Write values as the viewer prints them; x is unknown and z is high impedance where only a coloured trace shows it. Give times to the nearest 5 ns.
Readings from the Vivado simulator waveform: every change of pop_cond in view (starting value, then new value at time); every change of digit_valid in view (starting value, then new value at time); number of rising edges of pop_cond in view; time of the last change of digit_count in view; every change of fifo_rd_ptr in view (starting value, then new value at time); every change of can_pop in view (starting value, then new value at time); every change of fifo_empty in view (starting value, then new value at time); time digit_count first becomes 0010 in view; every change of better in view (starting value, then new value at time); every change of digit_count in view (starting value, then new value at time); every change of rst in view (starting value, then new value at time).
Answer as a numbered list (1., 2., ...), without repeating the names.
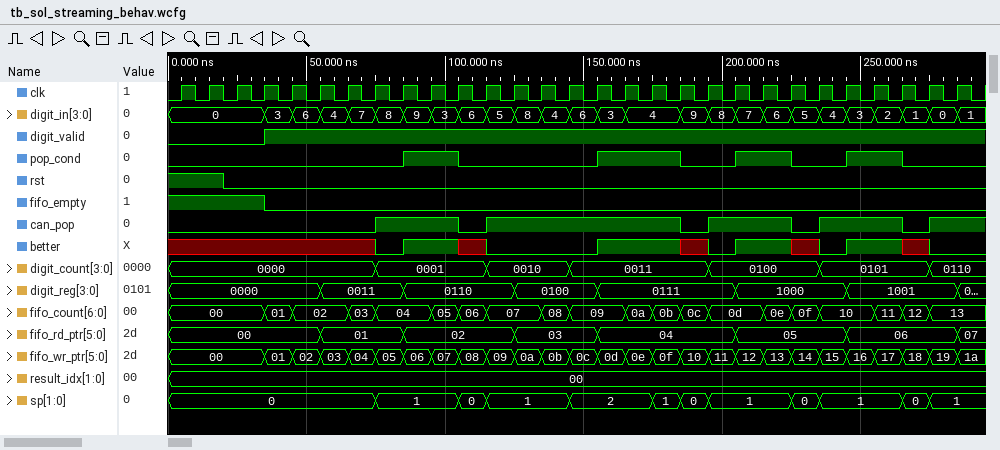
1. 0, 1 at 85 ns, 0 at 105 ns, 1 at 155 ns, 0 at 185 ns, 1 at 205 ns, 0 at 225 ns, 1 at 245 ns, 0 at 265 ns
2. 0, 1 at 35 ns
3. 4
4. 275 ns
5. 00, 01 at 55 ns, 02 at 85 ns, 03 at 125 ns, 04 at 155 ns, 05 at 205 ns, 06 at 245 ns, 07 at 285 ns
6. 0, 1 at 75 ns, 0 at 105 ns, 1 at 115 ns, 0 at 185 ns, 1 at 195 ns, 0 at 225 ns, 1 at 235 ns, 0 at 265 ns, 1 at 275 ns
7. 1, 0 at 35 ns
8. 115 ns
9. x, 0 at 75 ns, 1 at 85 ns, x at 105 ns, 0 at 115 ns, 1 at 155 ns, x at 185 ns, 0 at 195 ns, 1 at 205 ns, x at 225 ns, 0 at 235 ns, 1 at 245 ns, x at 265 ns, 0 at 275 ns
10. 0000, 0001 at 75 ns, 0010 at 115 ns, 0011 at 145 ns, 0100 at 195 ns, 0101 at 235 ns, 0110 at 275 ns
11. 1, 0 at 20 ns
